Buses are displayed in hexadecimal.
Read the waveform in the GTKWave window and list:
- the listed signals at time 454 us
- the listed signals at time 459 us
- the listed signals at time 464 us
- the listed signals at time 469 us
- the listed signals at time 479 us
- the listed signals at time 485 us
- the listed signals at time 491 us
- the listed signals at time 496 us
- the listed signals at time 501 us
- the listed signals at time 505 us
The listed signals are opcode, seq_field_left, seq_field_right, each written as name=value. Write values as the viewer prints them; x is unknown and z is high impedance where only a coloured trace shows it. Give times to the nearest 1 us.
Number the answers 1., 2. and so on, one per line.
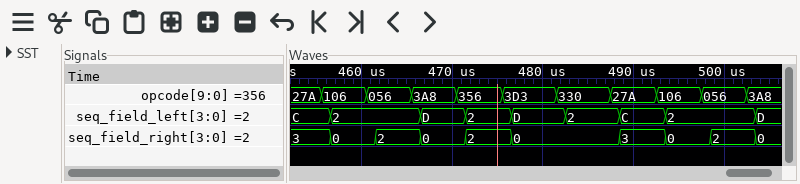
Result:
1. opcode=27A, seq_field_left=C, seq_field_right=3
2. opcode=106, seq_field_left=2, seq_field_right=0
3. opcode=056, seq_field_left=2, seq_field_right=2
4. opcode=3A8, seq_field_left=D, seq_field_right=0
5. opcode=3D3, seq_field_left=D, seq_field_right=0
6. opcode=330, seq_field_left=2, seq_field_right=0
7. opcode=27A, seq_field_left=C, seq_field_right=3
8. opcode=106, seq_field_left=2, seq_field_right=0
9. opcode=056, seq_field_left=2, seq_field_right=2
10. opcode=3A8, seq_field_left=D, seq_field_right=0
